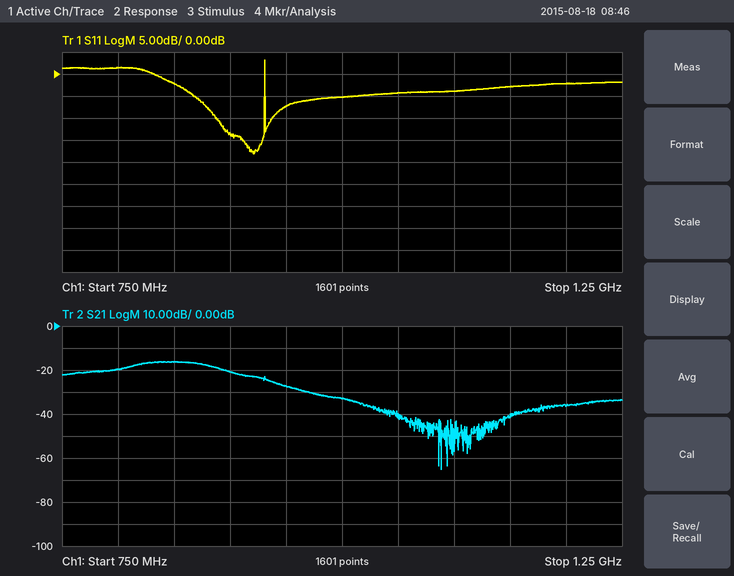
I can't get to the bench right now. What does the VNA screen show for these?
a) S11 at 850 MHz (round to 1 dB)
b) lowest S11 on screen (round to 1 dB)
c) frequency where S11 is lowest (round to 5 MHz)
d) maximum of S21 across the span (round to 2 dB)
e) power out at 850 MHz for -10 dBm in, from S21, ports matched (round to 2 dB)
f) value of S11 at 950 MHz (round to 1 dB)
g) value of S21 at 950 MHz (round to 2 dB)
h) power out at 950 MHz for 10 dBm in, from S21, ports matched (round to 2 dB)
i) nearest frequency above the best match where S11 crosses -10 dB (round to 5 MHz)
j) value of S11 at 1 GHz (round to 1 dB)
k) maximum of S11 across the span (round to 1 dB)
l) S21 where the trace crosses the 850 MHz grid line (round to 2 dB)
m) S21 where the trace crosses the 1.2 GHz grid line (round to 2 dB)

-2 dB
-18 dB
920 MHz
-16 dB
-26 dBm
-7 dB
-28 dB
-18 dBm
930 MHz
-5 dB
3 dB
-16 dB
-36 dB
